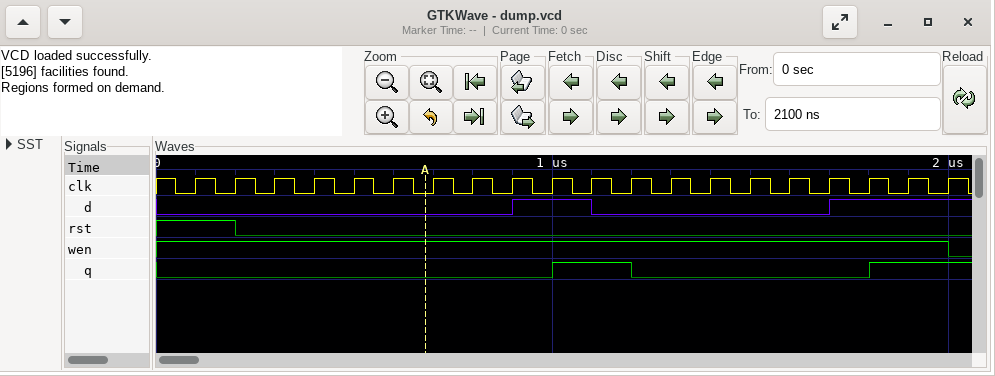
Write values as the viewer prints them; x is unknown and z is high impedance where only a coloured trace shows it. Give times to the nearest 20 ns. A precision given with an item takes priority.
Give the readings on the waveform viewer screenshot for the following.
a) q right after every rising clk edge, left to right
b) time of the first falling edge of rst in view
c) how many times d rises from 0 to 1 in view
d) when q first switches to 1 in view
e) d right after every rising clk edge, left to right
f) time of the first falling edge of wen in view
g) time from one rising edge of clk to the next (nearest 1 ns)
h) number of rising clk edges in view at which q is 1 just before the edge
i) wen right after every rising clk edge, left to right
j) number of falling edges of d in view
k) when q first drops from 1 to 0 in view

0 0 0 0 0 0 0 0 0 1 1 0 0 0 0 0 0 1 1 1
200 ns
2
1000 ns
0 0 0 0 0 0 0 0 1 1 0 0 0 0 0 0 1 1 1 1
2000 ns
100 ns
4
1 1 1 1 1 1 1 1 1 1 1 1 1 1 1 1 1 1 1 0
1
1200 ns
